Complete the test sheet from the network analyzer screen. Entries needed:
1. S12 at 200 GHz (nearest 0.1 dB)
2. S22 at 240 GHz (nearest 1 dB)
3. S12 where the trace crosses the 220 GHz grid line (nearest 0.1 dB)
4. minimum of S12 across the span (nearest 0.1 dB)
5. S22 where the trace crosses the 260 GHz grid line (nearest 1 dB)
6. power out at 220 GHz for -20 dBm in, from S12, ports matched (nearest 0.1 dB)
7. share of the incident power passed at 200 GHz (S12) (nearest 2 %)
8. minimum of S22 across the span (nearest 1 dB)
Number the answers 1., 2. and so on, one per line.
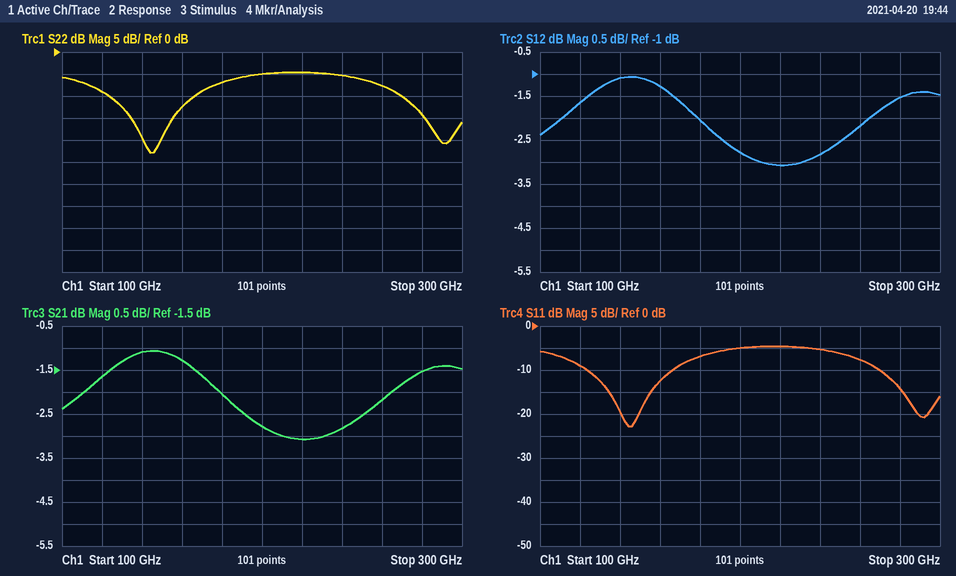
1. -2.8 dB
2. -5 dB
3. -3.1 dB
4. -3.1 dB
5. -8 dB
6. -23.1 dBm
7. 52 %
8. -23 dB
